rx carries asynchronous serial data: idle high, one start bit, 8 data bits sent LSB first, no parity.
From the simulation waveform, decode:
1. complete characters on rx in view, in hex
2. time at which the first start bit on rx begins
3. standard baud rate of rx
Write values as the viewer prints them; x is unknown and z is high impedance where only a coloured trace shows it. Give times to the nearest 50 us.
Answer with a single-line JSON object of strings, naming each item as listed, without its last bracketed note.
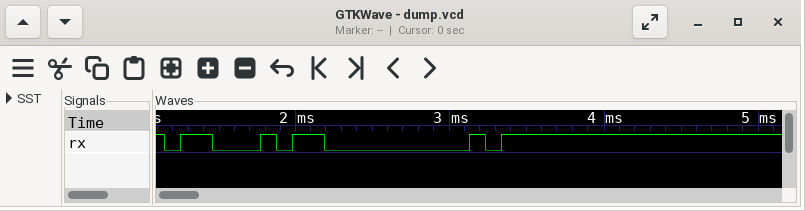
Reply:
{"complete characters on rx in view, in hex": "A3, 00, FF", "time at which the first start bit on rx begins": "1150 us", "standard baud rate of rx": "9600 baud"}
